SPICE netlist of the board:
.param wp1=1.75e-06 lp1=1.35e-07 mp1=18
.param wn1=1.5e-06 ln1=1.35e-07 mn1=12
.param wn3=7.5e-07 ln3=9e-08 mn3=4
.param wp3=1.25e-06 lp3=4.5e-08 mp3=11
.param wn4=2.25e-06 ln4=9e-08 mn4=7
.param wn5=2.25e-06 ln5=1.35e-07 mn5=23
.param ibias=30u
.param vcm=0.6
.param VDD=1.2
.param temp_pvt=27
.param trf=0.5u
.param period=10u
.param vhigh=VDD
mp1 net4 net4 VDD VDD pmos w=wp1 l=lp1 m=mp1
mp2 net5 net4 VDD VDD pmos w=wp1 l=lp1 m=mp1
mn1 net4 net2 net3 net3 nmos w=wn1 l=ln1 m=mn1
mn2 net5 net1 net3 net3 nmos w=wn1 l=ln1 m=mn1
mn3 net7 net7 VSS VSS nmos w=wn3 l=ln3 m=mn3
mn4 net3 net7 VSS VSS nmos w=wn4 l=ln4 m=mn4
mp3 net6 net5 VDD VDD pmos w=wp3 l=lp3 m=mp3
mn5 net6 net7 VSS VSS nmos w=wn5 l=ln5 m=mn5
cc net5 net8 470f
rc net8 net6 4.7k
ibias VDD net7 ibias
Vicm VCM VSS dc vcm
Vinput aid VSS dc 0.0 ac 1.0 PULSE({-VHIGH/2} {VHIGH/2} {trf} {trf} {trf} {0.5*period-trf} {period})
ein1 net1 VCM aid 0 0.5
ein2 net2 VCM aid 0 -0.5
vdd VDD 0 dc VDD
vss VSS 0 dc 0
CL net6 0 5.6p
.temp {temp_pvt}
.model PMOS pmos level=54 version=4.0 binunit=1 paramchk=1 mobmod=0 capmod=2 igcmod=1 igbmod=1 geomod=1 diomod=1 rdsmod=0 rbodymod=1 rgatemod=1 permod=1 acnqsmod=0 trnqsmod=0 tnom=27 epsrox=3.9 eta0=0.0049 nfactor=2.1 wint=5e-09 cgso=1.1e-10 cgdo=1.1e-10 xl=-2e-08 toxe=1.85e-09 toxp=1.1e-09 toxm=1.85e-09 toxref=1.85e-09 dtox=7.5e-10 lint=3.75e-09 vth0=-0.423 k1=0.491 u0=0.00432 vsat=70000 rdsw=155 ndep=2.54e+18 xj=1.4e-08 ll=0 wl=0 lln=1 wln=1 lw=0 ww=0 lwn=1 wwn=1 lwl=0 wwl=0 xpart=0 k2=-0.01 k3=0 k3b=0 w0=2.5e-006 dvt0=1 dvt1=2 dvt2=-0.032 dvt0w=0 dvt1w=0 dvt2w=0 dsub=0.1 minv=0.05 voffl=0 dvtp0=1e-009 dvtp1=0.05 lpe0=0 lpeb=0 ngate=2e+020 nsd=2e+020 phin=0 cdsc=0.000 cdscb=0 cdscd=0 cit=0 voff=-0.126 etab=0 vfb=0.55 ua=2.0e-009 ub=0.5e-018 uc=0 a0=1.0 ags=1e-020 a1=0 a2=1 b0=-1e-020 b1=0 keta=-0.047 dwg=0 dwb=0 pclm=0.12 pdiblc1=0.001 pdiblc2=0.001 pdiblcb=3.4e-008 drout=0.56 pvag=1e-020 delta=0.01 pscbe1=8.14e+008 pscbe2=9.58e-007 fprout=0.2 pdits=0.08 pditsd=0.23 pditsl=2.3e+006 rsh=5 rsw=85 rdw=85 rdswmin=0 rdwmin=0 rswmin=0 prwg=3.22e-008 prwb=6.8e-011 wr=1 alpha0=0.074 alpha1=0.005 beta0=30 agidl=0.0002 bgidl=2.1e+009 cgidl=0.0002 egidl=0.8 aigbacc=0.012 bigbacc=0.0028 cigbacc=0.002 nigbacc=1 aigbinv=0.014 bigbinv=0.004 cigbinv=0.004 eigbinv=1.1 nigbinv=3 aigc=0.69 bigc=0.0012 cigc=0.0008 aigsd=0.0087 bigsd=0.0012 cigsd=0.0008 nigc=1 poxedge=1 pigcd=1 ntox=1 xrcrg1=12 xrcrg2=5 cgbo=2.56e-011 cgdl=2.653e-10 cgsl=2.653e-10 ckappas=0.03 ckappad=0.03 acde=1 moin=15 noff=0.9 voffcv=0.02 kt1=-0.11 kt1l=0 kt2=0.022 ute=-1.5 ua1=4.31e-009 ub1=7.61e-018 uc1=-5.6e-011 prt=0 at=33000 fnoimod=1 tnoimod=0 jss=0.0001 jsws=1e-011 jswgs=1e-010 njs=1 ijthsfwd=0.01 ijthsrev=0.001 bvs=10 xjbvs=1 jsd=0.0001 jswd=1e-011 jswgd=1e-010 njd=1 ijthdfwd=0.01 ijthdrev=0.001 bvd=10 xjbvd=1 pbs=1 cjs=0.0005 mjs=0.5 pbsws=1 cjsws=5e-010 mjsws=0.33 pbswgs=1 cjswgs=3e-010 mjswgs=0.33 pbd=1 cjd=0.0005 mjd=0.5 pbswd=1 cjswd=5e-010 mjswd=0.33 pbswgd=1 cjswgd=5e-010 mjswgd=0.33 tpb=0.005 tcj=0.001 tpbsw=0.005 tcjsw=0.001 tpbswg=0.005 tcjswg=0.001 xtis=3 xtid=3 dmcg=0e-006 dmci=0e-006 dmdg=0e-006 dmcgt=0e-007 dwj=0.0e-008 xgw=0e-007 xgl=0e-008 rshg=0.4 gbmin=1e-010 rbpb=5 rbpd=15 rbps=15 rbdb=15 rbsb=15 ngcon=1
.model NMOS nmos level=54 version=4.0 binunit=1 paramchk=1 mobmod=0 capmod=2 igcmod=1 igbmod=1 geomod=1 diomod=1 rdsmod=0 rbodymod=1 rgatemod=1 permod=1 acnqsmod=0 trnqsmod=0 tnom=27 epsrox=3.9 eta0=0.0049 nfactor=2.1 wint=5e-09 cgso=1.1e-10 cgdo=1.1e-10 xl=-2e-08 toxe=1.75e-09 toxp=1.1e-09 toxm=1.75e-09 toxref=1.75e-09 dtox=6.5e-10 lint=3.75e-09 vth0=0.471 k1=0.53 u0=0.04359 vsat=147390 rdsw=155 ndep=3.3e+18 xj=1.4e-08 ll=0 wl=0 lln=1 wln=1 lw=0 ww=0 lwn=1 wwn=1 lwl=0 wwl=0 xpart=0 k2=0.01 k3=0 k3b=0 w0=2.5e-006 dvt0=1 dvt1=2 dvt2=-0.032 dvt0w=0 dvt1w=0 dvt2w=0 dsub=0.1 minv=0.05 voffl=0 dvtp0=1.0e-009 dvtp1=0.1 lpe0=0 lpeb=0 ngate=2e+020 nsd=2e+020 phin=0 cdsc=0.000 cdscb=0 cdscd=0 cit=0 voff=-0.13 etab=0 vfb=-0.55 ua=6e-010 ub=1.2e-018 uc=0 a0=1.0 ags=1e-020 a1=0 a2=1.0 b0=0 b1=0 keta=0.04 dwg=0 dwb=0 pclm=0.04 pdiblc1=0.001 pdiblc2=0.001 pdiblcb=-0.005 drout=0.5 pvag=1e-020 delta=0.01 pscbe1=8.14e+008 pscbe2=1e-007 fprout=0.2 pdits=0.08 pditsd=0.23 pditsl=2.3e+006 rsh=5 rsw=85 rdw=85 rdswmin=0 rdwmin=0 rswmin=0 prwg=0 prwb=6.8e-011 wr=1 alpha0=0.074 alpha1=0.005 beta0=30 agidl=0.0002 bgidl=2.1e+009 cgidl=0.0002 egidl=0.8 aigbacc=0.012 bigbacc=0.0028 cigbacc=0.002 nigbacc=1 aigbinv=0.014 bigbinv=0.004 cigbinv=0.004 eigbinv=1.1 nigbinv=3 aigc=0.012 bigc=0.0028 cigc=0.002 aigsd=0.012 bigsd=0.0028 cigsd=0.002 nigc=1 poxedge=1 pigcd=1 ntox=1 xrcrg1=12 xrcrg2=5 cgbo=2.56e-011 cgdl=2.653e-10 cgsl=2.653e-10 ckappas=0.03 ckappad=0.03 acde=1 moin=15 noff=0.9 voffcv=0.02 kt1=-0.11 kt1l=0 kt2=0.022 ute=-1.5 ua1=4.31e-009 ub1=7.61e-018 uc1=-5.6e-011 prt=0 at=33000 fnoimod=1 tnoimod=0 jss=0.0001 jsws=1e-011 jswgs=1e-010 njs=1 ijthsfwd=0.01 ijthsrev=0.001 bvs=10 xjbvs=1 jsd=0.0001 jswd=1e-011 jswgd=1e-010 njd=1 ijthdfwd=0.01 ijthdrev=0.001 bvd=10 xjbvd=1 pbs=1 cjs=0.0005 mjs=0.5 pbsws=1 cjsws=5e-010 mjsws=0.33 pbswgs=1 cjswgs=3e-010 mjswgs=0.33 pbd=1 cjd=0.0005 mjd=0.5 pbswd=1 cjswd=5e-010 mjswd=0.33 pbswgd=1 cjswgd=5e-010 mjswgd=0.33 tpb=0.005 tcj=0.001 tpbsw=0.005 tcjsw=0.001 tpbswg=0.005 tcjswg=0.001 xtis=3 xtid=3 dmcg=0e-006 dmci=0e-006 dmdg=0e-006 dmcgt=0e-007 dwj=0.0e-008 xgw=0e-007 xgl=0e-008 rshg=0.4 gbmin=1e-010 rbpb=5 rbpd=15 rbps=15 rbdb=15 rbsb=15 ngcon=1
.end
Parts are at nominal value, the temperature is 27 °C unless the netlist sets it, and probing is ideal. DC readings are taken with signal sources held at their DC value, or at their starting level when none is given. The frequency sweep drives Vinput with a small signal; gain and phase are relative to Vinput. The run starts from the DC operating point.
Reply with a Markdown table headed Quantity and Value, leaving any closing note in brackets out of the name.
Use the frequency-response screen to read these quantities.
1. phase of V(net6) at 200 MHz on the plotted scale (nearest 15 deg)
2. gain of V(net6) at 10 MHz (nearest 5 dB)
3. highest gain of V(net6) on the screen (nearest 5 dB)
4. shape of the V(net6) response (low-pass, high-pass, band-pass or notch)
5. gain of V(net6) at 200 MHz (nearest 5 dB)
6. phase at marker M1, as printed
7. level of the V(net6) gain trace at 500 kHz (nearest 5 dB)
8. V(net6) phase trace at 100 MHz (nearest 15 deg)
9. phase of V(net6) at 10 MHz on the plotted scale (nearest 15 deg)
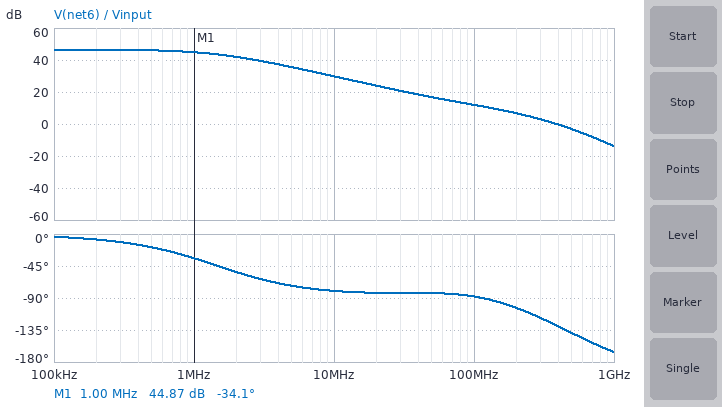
| Quantity | Value |
|---|---|
| phase of V(net6) at 200 MHz on the plotted scale | -105 deg |
| gain of V(net6) at 10 MHz | 30 dB |
| highest gain of V(net6) on the screen | 45 dB |
| shape of the V(net6) response | low-pass |
| gain of V(net6) at 200 MHz | 5 dB |
| phase at marker M1, as printed | -34.1 deg |
| level of the V(net6) gain trace at 500 kHz | 45 dB |
| V(net6) phase trace at 100 MHz | -90 deg |
| phase of V(net6) at 10 MHz on the plotted scale | -75 deg |
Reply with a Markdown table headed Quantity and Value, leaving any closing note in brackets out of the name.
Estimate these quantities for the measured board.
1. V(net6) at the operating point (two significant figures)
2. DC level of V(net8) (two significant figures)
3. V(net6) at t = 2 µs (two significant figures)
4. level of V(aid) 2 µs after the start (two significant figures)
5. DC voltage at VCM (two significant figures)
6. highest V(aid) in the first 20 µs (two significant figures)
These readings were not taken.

| Quantity | Value |
|---|---|
| V(net6) at the operating point | 1.0 V |
| DC level of V(net8) | 1.0 V |
| V(net6) at t = 2 µs | 1.2 V |
| level of V(aid) 2 µs after the start | 600 mV |
| DC voltage at VCM | 600 mV |
| highest V(aid) in the first 20 µs | 600 mV |
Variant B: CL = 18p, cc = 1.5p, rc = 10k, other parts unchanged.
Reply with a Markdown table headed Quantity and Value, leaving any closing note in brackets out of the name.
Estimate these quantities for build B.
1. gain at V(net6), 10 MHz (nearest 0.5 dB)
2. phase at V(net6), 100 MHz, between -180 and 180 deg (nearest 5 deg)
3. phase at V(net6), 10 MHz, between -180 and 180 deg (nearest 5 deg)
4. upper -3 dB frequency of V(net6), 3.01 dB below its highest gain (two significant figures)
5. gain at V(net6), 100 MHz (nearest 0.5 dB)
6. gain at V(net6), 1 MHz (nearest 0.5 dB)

| Quantity | Value |
|---|---|
| gain at V(net6), 10 MHz | 22.0 dB |
| phase at V(net6), 100 MHz, between -180 and 180 deg | -100 deg |
| phase at V(net6), 10 MHz, between -180 and 180 deg | -60 deg |
| upper -3 dB frequency of V(net6), 3.01 dB below its highest gain | 460 kHz |
| gain at V(net6), 100 MHz | 9.5 dB |
| gain at V(net6), 1 MHz | 39.0 dB |
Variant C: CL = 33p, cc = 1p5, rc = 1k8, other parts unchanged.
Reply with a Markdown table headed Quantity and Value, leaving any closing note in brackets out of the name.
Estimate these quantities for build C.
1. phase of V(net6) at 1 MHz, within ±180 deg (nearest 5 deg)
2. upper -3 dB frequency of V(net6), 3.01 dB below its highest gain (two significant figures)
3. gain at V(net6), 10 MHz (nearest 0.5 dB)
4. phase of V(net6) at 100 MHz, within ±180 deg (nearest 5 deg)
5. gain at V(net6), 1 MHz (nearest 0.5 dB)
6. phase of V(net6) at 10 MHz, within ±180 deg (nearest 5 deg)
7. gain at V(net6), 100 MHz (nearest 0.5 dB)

| Quantity | Value |
|---|---|
| phase of V(net6) at 1 MHz, within ±180 deg | -65 deg |
| upper -3 dB frequency of V(net6), 3.01 dB below its highest gain | 460 kHz |
| gain at V(net6), 10 MHz | 19.0 dB |
| phase of V(net6) at 100 MHz, within ±180 deg | -120 deg |
| gain at V(net6), 1 MHz | 39.0 dB |
| phase of V(net6) at 10 MHz, within ±180 deg | -105 deg |
| gain at V(net6), 100 MHz | -8.5 dB |
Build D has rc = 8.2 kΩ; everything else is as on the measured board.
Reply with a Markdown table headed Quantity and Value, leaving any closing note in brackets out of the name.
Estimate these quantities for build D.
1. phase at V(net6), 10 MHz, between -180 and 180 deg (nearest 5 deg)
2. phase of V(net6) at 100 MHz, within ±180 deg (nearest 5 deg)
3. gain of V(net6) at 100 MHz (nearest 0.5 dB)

| Quantity | Value |
|---|---|
| phase at V(net6), 10 MHz, between -180 and 180 deg | -75 deg |
| phase of V(net6) at 100 MHz, within ±180 deg | -80 deg |
| gain of V(net6) at 100 MHz | 15.5 dB |
